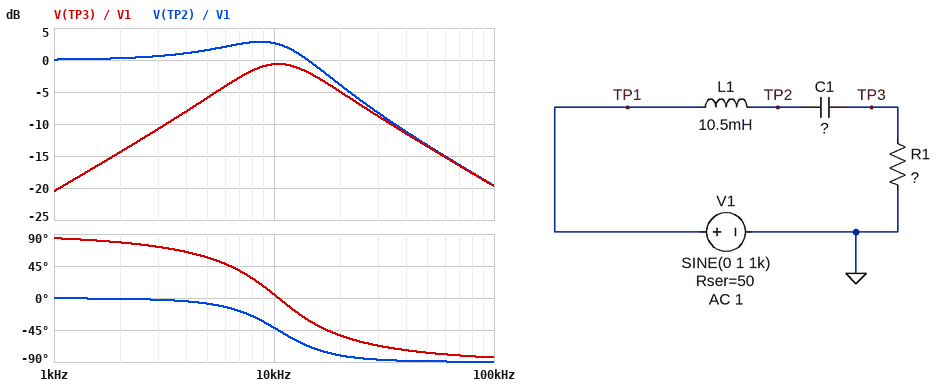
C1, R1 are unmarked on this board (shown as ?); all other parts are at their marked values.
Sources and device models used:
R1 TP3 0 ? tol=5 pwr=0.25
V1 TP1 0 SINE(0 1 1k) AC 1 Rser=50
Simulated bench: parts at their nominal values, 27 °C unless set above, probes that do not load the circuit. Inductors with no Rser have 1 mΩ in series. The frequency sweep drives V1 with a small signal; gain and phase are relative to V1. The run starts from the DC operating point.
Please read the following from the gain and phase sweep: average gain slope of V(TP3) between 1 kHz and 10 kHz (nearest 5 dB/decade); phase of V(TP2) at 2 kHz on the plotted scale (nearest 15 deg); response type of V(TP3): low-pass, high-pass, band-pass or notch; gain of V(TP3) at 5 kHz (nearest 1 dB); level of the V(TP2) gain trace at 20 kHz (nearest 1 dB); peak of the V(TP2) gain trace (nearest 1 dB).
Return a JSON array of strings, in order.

["20 dB/decade", "0 deg", "band-pass", "-6 dB", "-4 dB", "3 dB"]
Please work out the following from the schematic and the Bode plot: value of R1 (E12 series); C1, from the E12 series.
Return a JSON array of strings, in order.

["680 Ω", "22 nF"]
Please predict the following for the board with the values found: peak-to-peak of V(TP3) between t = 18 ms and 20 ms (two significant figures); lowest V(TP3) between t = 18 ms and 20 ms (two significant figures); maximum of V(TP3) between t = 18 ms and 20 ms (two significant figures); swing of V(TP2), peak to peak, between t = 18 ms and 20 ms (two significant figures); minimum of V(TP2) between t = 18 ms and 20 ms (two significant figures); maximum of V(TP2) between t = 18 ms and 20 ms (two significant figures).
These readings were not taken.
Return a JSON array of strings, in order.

["190 mV", "-94 mV", "94 mV", "2.0 V", "-1.0 V", "1.0 V"]
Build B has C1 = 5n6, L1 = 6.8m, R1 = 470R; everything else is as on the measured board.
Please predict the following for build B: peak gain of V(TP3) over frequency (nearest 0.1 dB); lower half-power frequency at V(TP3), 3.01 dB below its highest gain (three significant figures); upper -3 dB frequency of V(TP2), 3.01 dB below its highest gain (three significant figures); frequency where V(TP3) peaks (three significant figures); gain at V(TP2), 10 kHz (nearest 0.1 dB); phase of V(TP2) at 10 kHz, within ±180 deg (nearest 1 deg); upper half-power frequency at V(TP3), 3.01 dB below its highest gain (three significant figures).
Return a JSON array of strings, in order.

["-0.9 dB", "20.4 kHz", "30.3 kHz", "25.8 kHz", "1.3 dB", "-3 deg", "32.6 kHz"]
